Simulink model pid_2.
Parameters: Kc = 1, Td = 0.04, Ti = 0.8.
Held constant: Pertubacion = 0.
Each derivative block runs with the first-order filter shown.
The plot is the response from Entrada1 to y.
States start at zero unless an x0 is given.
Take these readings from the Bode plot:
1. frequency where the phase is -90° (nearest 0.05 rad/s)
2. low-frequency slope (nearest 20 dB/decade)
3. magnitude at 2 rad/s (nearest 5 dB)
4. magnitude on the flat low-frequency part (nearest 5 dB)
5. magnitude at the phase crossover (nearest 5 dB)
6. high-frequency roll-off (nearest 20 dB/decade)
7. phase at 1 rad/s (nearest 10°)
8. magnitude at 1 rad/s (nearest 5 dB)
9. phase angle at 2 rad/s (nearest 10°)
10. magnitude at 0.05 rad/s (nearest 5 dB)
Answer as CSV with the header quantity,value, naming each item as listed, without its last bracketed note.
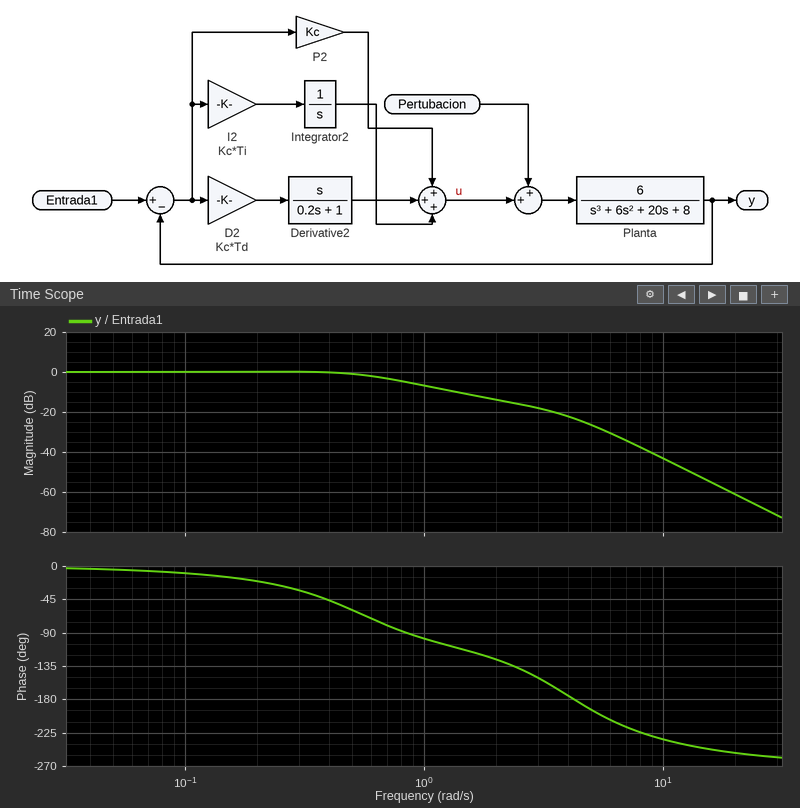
quantity,value
frequency where the phase is -90°,0.85 rad/s
low-frequency slope,0 dB/decade
magnitude at 2 rad/s,-15 dB
magnitude on the flat low-frequency part,0 dB
magnitude at the phase crossover,-25 dB
high-frequency roll-off,-60 dB/decade
phase at 1 rad/s,-100°
magnitude at 1 rad/s,-5 dB
phase angle at 2 rad/s,-130°
magnitude at 0.05 rad/s,0 dB
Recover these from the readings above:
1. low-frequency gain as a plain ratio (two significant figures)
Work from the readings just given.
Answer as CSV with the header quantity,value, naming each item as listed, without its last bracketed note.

quantity,value
low-frequency gain as a plain ratio,1.0
